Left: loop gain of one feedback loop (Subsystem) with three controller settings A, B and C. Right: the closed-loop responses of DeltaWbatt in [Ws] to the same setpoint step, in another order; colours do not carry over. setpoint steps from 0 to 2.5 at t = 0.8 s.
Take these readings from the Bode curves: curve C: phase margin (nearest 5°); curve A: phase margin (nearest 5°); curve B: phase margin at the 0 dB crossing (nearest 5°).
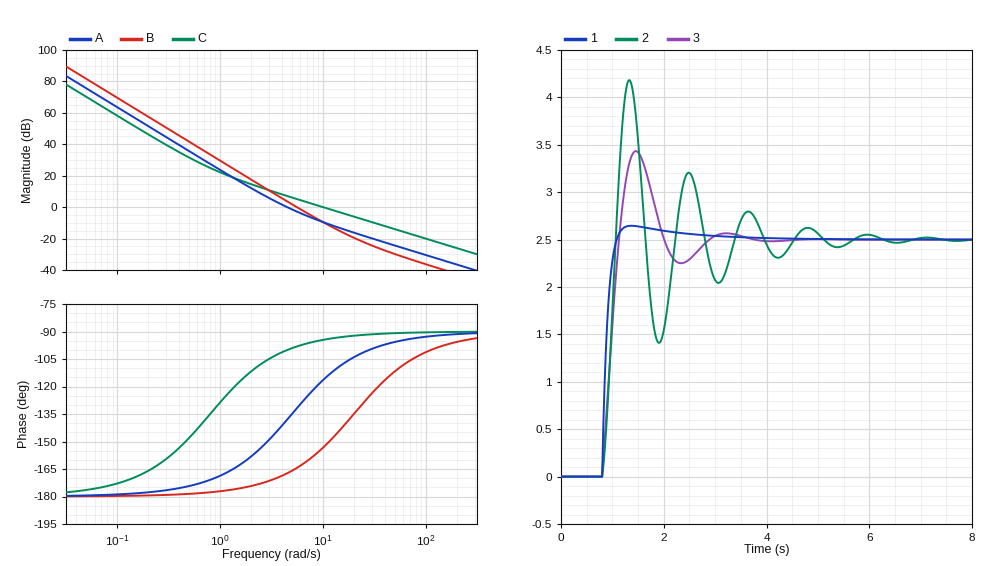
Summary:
85°
40°
15°
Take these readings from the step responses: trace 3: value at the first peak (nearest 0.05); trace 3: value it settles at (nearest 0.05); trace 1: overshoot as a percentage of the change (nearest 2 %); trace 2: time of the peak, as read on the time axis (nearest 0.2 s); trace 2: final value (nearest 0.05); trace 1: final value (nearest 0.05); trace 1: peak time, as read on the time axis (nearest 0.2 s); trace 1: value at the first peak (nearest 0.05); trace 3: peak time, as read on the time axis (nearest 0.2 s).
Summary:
3.45
2.50
6 %
1.4 s
2.50
2.50
1.4 s
2.65
1.4 s
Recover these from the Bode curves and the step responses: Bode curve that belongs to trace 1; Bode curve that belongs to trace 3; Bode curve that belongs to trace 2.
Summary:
C
A
B
